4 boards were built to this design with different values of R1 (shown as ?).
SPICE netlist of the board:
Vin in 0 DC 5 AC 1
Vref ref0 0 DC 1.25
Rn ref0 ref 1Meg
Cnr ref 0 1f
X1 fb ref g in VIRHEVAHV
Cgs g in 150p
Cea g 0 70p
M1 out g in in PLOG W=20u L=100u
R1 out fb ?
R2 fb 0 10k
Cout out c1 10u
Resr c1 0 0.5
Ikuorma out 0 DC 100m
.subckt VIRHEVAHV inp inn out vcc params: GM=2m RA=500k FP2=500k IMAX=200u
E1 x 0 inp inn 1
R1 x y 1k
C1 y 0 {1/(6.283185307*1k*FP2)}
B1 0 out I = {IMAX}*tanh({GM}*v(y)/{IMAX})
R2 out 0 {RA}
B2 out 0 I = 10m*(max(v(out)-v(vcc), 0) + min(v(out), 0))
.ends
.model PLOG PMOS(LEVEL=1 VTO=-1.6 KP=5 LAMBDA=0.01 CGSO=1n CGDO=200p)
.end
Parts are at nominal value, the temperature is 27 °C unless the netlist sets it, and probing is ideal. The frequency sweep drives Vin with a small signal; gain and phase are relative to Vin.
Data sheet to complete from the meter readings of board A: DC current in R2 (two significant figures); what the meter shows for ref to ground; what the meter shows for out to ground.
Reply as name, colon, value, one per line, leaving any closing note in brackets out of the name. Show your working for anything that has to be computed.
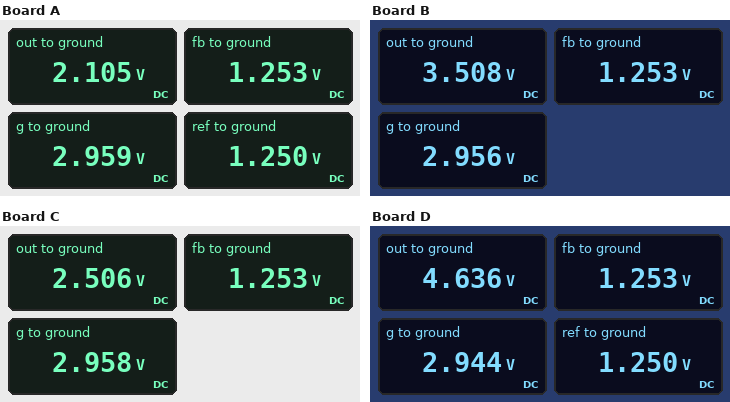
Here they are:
DC current in R2: (1.253 V) / 10 kΩ = 130 µA
what the meter shows for ref to ground: 1.250 V
what the meter shows for out to ground: 2.105 V
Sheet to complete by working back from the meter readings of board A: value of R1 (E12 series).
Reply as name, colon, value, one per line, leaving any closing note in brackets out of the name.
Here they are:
value of R1: 6.8 kΩ
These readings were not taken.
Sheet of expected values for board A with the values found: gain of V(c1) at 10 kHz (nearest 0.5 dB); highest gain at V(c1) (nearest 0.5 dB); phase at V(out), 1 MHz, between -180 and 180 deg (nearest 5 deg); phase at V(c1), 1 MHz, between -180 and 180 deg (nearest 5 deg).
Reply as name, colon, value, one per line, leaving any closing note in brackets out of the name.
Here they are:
gain of V(c1) at 10 kHz: -58.0 dB
highest gain at V(c1): -20.5 dB
phase at V(out), 1 MHz, between -180 and 180 deg: 0 deg
phase at V(c1), 1 MHz, between -180 and 180 deg: 0 deg
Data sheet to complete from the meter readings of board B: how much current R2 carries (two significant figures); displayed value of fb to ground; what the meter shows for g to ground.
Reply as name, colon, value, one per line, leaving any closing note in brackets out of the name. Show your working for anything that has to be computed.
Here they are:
how much current R2 carries: (1.253 V) / 10 kΩ = 130 µA
displayed value of fb to ground: 1.253 V
what the meter shows for g to ground: 2.956 V
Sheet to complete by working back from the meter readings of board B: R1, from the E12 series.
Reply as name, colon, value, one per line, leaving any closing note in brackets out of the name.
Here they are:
R1, from the E12 series: 18 kΩ
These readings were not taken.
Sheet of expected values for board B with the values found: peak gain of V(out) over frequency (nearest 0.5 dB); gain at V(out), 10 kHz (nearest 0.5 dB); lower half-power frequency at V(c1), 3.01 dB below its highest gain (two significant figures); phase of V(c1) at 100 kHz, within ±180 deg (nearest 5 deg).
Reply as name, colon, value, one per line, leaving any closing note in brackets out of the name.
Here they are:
peak gain of V(out) over frequency: -21.5 dB
gain at V(out), 10 kHz: -43.0 dB
lower half-power frequency at V(c1), 3.01 dB below its highest gain: 94 kHz
phase of V(c1) at 100 kHz, within ±180 deg: 65 deg
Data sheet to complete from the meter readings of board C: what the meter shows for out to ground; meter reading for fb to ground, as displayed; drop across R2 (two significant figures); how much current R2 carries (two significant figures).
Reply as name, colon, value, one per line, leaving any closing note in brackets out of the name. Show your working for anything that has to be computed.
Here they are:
what the meter shows for out to ground: 2.506 V
meter reading for fb to ground, as displayed: 1.253 V
drop across R2: 1.253 V = 1.3 V
how much current R2 carries: (1.253 V) / 10 kΩ = 130 µA
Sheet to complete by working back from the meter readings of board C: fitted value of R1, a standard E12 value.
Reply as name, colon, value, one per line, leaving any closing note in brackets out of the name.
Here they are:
fitted value of R1, a standard E12 value: 10 kΩ
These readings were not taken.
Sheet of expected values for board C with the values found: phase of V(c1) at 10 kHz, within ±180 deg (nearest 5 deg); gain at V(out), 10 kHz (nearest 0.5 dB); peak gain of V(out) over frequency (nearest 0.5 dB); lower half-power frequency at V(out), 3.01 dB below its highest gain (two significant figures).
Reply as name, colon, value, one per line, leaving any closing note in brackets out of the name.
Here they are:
phase of V(c1) at 10 kHz, within ±180 deg: 140 deg
gain at V(out), 10 kHz: -46.0 dB
peak gain of V(out) over frequency: -21.0 dB
lower half-power frequency at V(out), 3.01 dB below its highest gain: 130 kHz
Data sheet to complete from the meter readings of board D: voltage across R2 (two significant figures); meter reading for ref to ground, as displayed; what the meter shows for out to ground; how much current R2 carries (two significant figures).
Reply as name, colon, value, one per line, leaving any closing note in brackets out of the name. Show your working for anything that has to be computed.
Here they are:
voltage across R2: 1.253 V = 1.3 V
meter reading for ref to ground, as displayed: 1.250 V
what the meter shows for out to ground: 4.636 V
how much current R2 carries: (1.253 V) / 10 kΩ = 130 µA
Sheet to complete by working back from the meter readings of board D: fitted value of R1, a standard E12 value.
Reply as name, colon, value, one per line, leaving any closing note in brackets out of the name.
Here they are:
fitted value of R1, a standard E12 value: 27 kΩ
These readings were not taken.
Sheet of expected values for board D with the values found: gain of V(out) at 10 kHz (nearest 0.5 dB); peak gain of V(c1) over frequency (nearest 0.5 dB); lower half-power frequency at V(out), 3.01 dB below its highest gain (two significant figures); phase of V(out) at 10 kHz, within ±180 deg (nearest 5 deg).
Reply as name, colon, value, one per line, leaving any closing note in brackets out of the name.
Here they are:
gain of V(out) at 10 kHz: -36.0 dB
peak gain of V(c1) over frequency: -19.0 dB
lower half-power frequency at V(out), 3.01 dB below its highest gain: 44 kHz
phase of V(out) at 10 kHz, within ±180 deg: 70 deg
